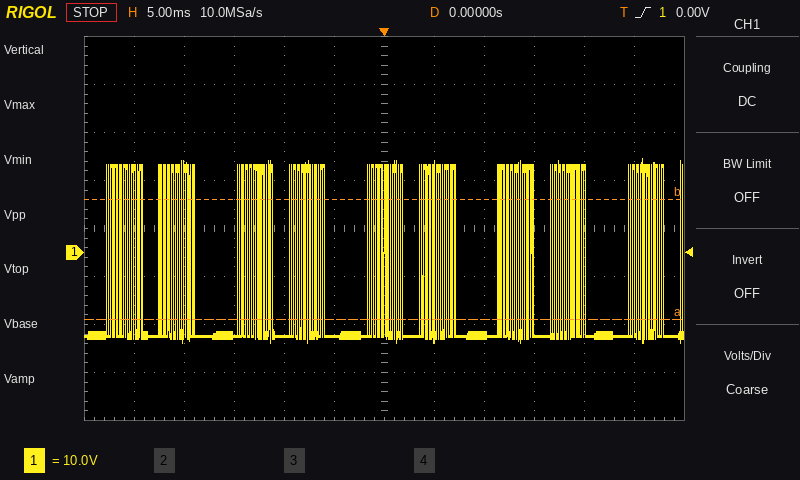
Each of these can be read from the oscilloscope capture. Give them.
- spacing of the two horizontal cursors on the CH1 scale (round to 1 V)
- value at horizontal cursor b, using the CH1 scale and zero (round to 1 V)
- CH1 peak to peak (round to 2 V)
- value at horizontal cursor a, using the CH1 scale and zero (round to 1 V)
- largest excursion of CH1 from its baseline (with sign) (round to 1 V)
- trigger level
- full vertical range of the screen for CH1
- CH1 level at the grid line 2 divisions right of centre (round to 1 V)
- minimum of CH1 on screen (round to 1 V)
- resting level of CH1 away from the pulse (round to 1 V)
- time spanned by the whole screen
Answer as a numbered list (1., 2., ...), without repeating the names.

1. 25 V
2. 11 V
3. 38 V
4. -14 V
5. +37 V
6. 0.00 V
7. 80 V
8. -17 V
9. -19 V
10. -17 V
11. 60 ms
